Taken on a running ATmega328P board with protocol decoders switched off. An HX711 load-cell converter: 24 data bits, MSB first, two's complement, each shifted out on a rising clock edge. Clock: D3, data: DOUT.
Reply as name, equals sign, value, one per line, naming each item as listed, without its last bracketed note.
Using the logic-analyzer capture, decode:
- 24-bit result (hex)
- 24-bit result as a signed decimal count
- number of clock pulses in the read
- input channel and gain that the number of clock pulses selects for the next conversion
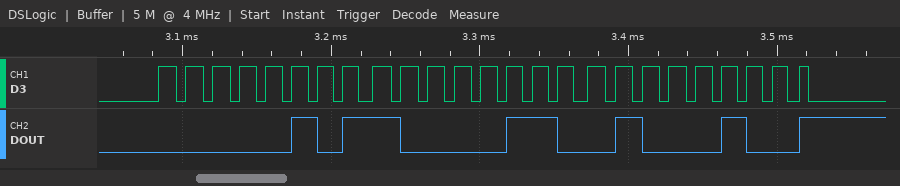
24-bit result = 0x058644
24-bit result as a signed decimal count = 362052
number of clock pulses in the read = 25
input channel and gain that the number of clock pulses selects for the next conversion = channel A, gain 128
